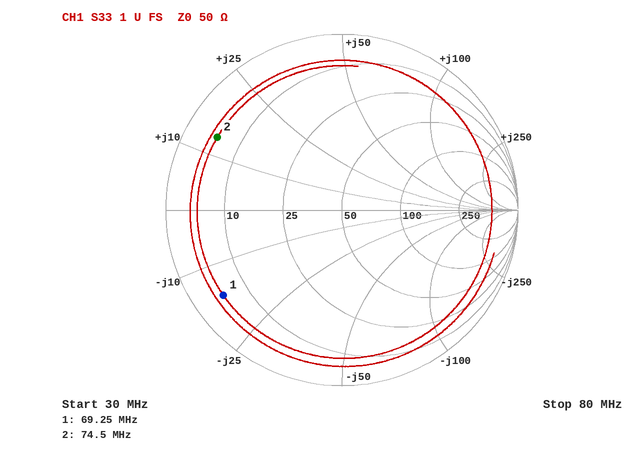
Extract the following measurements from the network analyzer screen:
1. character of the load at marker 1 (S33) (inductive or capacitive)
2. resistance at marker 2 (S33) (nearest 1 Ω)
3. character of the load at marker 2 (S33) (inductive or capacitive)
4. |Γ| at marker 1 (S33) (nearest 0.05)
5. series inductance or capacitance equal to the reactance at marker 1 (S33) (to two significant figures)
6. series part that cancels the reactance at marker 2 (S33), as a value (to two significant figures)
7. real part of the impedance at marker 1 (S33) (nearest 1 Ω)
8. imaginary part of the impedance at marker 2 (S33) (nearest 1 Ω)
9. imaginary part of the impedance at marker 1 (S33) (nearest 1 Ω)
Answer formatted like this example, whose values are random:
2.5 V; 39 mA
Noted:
capacitive; 5 Ω; inductive; 0.85; 140 pF; 160 pF; 5 Ω; +13 Ω; -16 Ω
